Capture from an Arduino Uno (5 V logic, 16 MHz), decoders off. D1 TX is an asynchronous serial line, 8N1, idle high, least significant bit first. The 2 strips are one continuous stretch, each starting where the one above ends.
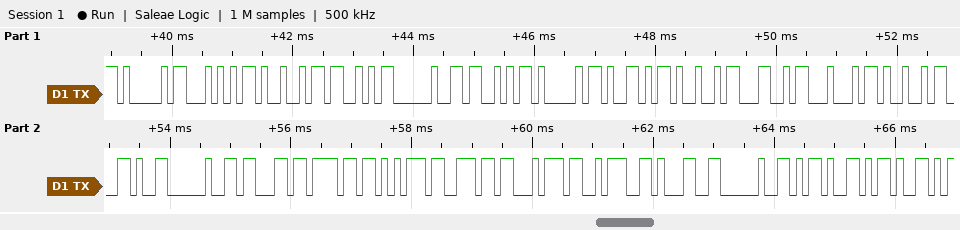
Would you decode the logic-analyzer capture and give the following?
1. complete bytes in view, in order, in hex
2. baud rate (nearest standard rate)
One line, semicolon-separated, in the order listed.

41 54 49 53 20 53 41 59 49 4C 44 49 2C 20 63 6F 75 6E 74 3A 31 20 2D 2D; 9600 baud
